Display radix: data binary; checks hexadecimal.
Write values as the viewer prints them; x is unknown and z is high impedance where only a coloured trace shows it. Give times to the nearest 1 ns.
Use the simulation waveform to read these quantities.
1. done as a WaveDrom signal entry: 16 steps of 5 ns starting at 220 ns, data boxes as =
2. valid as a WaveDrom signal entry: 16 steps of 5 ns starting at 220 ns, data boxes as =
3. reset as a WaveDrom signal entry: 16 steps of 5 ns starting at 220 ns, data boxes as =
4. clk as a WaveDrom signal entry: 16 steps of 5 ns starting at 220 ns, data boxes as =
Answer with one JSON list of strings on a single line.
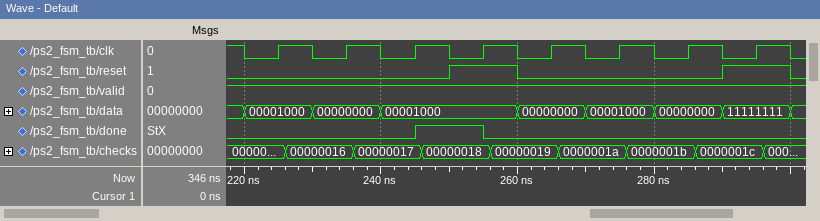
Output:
["{name: 'done', wave: '0....1.0........'}", "{name: 'valid', wave: '1...............'}", "{name: 'reset', wave: '0.....1.0.....1.'}", "{name: 'clk', wave: '0101010101010101'}"]
